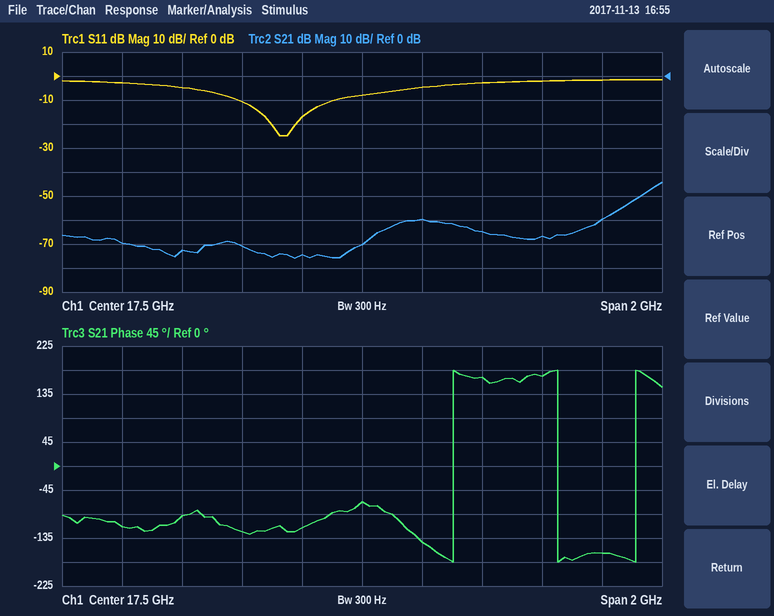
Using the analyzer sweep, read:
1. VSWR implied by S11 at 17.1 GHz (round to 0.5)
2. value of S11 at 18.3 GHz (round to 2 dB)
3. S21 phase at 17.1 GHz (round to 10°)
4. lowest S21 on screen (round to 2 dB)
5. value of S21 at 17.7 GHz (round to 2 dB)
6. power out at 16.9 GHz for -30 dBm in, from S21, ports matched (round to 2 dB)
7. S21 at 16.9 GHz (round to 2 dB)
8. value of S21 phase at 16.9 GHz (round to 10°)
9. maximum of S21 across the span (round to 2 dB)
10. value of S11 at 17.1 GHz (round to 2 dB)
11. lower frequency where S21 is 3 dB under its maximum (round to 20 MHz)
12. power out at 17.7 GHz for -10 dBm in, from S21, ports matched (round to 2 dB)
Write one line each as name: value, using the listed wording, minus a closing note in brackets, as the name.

VSWR implied by S11 at 17.1 GHz: 2.0
value of S11 at 18.3 GHz: -2 dB
S21 phase at 17.1 GHz: -120°
lowest S21 on screen: -76 dB
value of S21 at 17.7 GHz: -60 dB
power out at 16.9 GHz for -30 dBm in, from S21, ports matched: -102 dBm
S21 at 16.9 GHz: -72 dB
value of S21 phase at 16.9 GHz: -90°
maximum of S21 across the span: -44 dB
value of S11 at 17.1 GHz: -10 dB
lower frequency where S21 is 3 dB under its maximum: 18.46 GHz
power out at 17.7 GHz for -10 dBm in, from S21, ports matched: -70 dBm
